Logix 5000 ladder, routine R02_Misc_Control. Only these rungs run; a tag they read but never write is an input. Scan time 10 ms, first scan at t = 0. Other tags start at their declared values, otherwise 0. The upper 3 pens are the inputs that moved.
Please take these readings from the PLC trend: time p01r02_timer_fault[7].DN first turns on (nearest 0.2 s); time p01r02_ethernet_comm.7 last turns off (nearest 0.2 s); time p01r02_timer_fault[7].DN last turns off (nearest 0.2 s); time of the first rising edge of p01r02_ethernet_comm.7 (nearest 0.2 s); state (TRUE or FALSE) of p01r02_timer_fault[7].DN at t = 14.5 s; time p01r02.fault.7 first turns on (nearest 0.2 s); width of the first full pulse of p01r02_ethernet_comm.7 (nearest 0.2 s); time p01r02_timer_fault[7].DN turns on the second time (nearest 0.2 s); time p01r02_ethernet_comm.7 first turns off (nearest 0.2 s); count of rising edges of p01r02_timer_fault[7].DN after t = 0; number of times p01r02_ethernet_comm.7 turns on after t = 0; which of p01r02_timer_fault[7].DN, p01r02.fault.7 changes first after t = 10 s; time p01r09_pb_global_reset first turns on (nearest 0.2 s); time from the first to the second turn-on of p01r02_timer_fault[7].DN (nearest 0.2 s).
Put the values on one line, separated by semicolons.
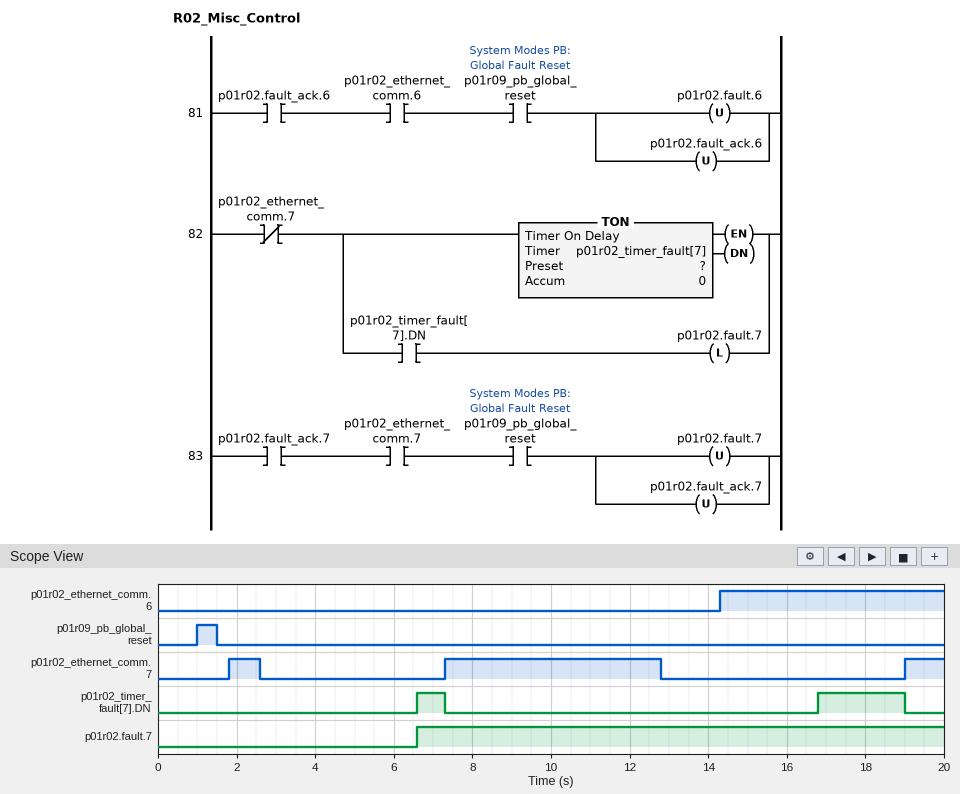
6.6 s; 12.8 s; 19.0 s; 1.8 s; FALSE; 6.6 s; 0.8 s; 16.8 s; 2.6 s; 2; 3; p01r02_timer_fault[7].DN; 1.0 s; 10.2 s
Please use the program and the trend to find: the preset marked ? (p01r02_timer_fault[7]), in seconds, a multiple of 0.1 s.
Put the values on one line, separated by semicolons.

4.0 s
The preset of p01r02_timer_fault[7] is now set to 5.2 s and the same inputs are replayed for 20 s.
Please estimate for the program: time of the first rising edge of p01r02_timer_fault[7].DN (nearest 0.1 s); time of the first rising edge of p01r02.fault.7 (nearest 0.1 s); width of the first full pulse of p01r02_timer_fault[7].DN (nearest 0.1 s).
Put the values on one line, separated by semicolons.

18.0 s; 18.0 s; 1.0 s
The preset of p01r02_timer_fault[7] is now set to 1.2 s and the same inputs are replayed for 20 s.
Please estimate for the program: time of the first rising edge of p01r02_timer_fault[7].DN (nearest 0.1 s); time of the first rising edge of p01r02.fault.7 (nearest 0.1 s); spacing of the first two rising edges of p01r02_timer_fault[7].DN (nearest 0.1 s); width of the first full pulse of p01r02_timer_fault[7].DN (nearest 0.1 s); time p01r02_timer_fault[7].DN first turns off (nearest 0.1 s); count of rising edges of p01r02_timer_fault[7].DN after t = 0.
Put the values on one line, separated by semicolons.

1.2 s; 1.2 s; 2.6 s; 0.6 s; 1.8 s; 3
